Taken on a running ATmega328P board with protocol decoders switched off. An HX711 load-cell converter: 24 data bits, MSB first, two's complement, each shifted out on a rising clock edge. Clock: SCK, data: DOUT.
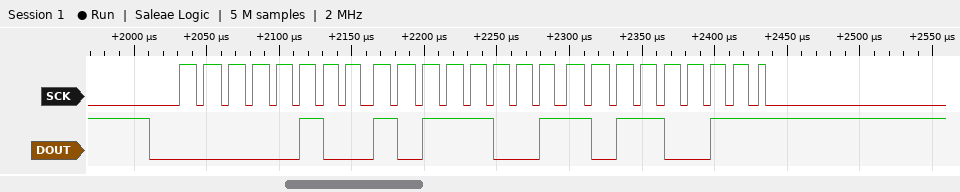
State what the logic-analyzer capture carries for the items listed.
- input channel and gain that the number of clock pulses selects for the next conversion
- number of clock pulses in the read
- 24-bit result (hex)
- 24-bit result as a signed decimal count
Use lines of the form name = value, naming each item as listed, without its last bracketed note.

input channel and gain that the number of clock pulses selects for the next conversion = channel A, gain 128
number of clock pulses in the read = 25
24-bit result = 0x04B9B3
24-bit result as a signed decimal count = 309683
